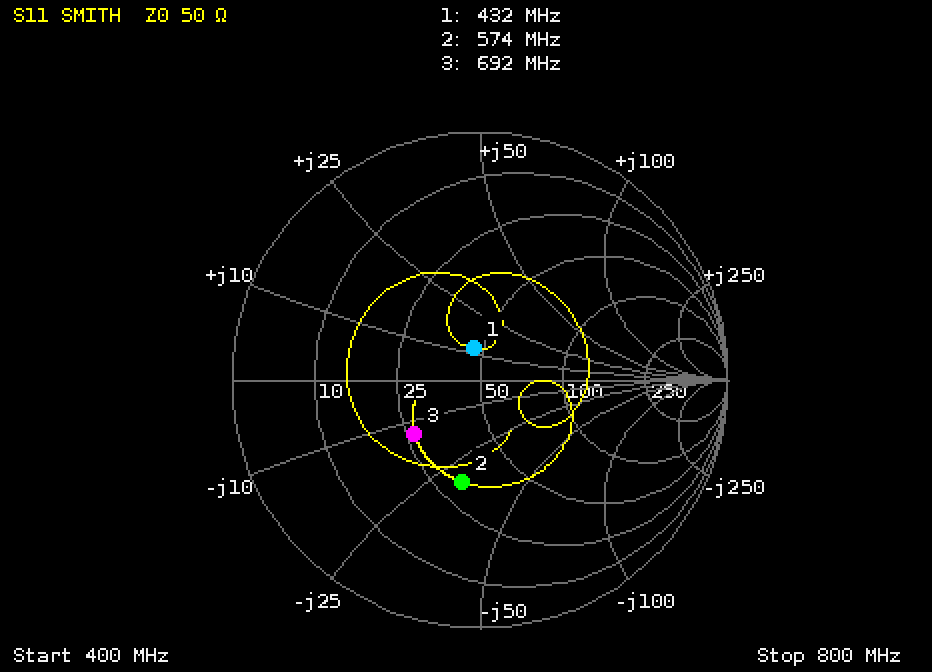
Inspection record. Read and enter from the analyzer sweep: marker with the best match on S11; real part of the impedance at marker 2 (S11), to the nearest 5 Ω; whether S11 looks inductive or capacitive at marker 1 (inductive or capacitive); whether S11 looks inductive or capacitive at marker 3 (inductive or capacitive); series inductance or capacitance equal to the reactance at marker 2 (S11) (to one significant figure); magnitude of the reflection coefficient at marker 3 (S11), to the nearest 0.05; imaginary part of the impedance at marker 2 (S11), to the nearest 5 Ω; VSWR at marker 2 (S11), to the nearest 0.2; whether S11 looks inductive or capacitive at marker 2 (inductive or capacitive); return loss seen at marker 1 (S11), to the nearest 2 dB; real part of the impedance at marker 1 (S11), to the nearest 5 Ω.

marker 1
30 Ω
inductive
capacitive
9 pF
0.35
-30 Ω
2.4
capacitive
18 dB
45 Ω
